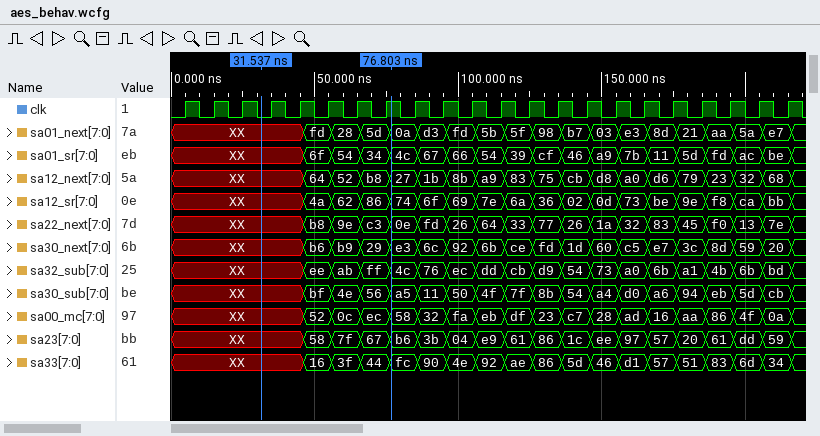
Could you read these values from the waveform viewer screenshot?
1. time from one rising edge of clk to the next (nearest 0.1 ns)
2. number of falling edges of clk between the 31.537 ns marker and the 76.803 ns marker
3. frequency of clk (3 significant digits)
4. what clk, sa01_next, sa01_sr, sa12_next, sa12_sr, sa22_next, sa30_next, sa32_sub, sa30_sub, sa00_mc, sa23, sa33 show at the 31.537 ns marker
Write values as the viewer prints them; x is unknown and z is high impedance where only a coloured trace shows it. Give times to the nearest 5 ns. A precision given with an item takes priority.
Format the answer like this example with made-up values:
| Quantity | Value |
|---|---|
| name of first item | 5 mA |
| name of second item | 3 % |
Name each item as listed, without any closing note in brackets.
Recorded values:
| Quantity | Value |
|---|---|
| time from one rising edge of clk to the next | 10 ns |
| number of falling edges of clk between the 31.537 ns marker and the 76.803 ns marker | 4 |
| frequency of clk | 100 MHz |
| what clk, sa01_next, sa01_sr, sa12_next, sa12_sr, sa22_next, sa30_next, sa32_sub, sa30_sub, sa00_mc, sa23, sa33 show at the 31.537 ns marker | clk=0, sa01_next=XX, sa01_sr=XX, sa12_next=XX, sa12_sr=XX, sa22_next=XX, sa30_next=XX, sa32_sub=XX, sa30_sub=XX, sa00_mc=XX, sa23=XX, sa33=XX |
